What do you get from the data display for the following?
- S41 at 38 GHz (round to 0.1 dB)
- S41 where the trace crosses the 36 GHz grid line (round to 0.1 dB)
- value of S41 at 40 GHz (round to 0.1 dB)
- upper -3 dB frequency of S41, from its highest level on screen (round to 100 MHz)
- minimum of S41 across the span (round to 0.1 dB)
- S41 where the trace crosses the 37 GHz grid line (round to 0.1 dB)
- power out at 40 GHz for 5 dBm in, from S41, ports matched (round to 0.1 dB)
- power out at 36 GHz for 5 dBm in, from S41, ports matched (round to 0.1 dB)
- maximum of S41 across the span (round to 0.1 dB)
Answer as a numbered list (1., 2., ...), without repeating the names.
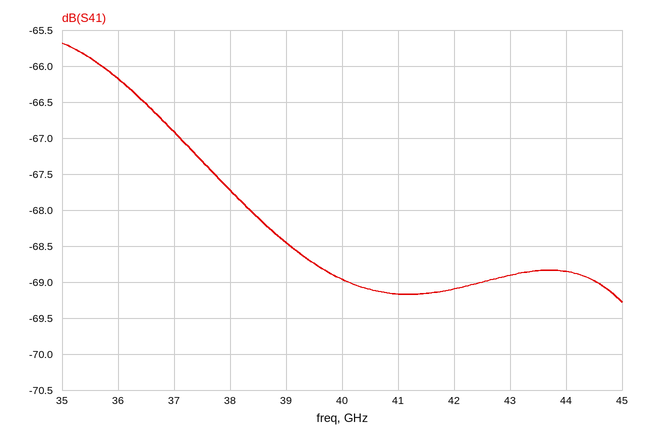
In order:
1. -67.7 dB
2. -66.2 dB
3. -69.0 dB
4. 39.4 GHz
5. -69.3 dB
6. -66.9 dB
7. -64.0 dBm
8. -61.2 dBm
9. -65.7 dB
